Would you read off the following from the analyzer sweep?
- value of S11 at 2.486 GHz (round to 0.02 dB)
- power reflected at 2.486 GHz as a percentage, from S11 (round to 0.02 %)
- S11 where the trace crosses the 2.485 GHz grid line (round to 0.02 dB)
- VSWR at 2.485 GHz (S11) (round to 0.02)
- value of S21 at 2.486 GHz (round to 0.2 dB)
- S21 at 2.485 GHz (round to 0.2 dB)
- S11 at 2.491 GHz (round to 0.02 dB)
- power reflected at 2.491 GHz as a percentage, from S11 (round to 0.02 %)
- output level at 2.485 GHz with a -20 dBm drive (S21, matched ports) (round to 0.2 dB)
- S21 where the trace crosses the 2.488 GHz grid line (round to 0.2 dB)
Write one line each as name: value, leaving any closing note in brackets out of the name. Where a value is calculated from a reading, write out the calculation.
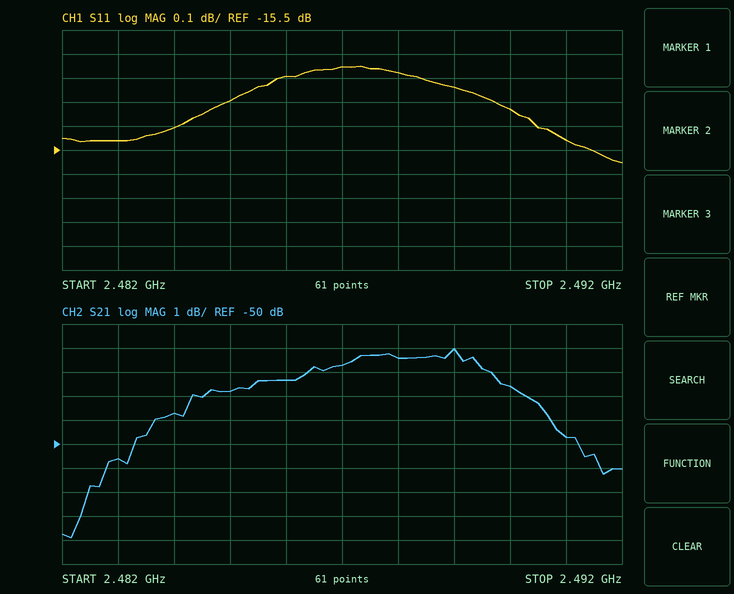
value of S11 at 2.486 GHz: -15.20 dB
power reflected at 2.486 GHz as a percentage, from S11: 10^(-15.2/10) ≈ 3.02 %
S11 where the trace crosses the 2.485 GHz grid line: -15.30 dB
VSWR at 2.485 GHz (S11): |Γ| = 10^(-15.3/20) = 0.1718; VSWR = (1 + 0.1718)/(1 − 0.1718) ≈ 1.41, so 1.42 to the nearest 0.02
value of S21 at 2.486 GHz: -47.4 dB
S21 at 2.485 GHz: -47.8 dB
S11 at 2.491 GHz: -15.46 dB
power reflected at 2.491 GHz as a percentage, from S11: 10^(-15.46/10) ≈ 2.84 %
output level at 2.485 GHz with a -20 dBm drive (S21, matched ports): -20 dBm + (-47.8 dB) = -67.8 dBm
S21 where the trace crosses the 2.488 GHz grid line: -46.4 dB
